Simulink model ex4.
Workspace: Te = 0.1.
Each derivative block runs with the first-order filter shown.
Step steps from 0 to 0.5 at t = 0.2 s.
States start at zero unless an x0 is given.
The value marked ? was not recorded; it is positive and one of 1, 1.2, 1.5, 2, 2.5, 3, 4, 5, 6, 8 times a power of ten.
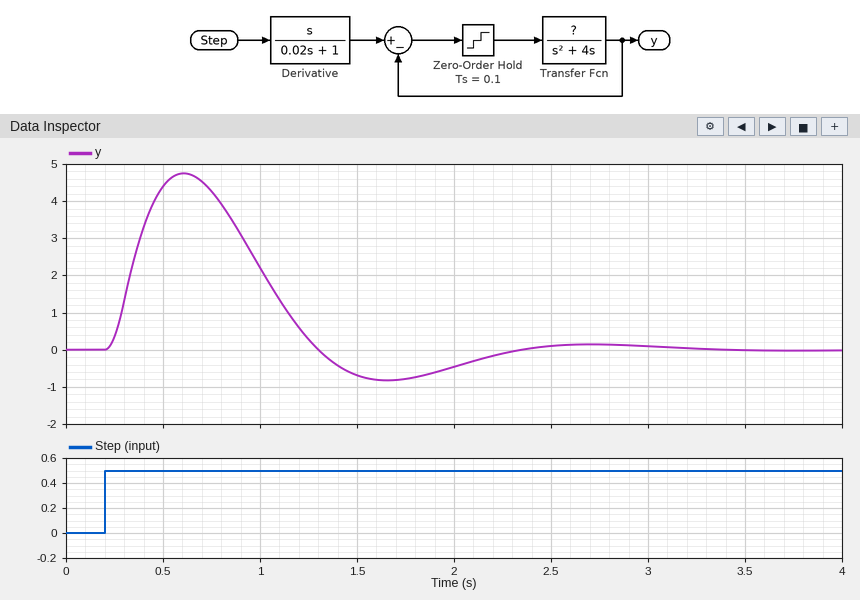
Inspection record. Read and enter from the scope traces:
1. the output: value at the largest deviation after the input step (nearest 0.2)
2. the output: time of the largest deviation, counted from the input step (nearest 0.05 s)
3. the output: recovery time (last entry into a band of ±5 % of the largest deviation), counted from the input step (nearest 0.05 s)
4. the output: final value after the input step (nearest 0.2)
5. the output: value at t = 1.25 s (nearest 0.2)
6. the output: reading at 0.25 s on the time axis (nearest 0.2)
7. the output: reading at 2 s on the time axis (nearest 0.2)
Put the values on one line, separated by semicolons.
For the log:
4.8; 0.40 s; 1.95 s; 0.0; 0.2; 0.4; -0.4
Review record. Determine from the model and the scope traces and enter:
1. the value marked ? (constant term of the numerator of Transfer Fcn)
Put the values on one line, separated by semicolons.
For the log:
12
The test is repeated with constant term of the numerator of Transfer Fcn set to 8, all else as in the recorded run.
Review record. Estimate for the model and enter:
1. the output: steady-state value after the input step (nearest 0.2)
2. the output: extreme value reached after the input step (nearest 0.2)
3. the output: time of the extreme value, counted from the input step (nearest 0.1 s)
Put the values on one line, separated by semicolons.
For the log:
0.0; 3.4; 0.5 s
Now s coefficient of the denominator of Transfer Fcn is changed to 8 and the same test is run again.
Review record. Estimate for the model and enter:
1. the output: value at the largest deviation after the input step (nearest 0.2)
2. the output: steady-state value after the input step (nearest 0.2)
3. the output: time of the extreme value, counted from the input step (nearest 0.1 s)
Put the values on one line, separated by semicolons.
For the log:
3.0; 0.0; 0.3 s
